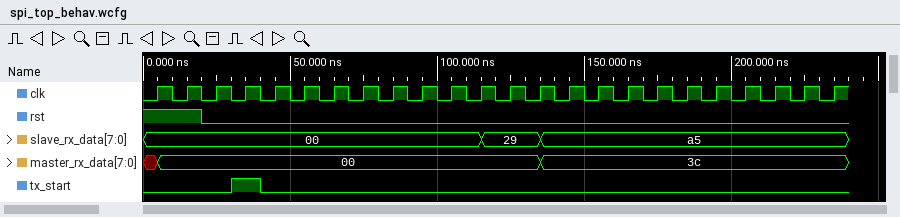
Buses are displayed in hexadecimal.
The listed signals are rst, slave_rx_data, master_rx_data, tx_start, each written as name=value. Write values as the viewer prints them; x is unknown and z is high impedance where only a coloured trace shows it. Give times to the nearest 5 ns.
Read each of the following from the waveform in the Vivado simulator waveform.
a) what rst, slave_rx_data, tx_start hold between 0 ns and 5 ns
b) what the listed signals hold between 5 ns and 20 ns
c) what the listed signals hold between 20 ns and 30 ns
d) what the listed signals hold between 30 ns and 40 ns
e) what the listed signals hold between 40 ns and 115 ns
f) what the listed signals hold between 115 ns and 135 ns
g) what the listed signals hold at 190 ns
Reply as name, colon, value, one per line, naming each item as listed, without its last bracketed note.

what rst, slave_rx_data, tx_start hold between 0 ns and 5 ns: rst=1, slave_rx_data=00, tx_start=0
what the listed signals hold between 5 ns and 20 ns: rst=1, slave_rx_data=00, master_rx_data=00, tx_start=0
what the listed signals hold between 20 ns and 30 ns: rst=0, slave_rx_data=00, master_rx_data=00, tx_start=0
what the listed signals hold between 30 ns and 40 ns: rst=0, slave_rx_data=00, master_rx_data=00, tx_start=1
what the listed signals hold between 40 ns and 115 ns: rst=0, slave_rx_data=00, master_rx_data=00, tx_start=0
what the listed signals hold between 115 ns and 135 ns: rst=0, slave_rx_data=29, master_rx_data=00, tx_start=0
what the listed signals hold at 190 ns: rst=0, slave_rx_data=a5, master_rx_data=3c, tx_start=0
